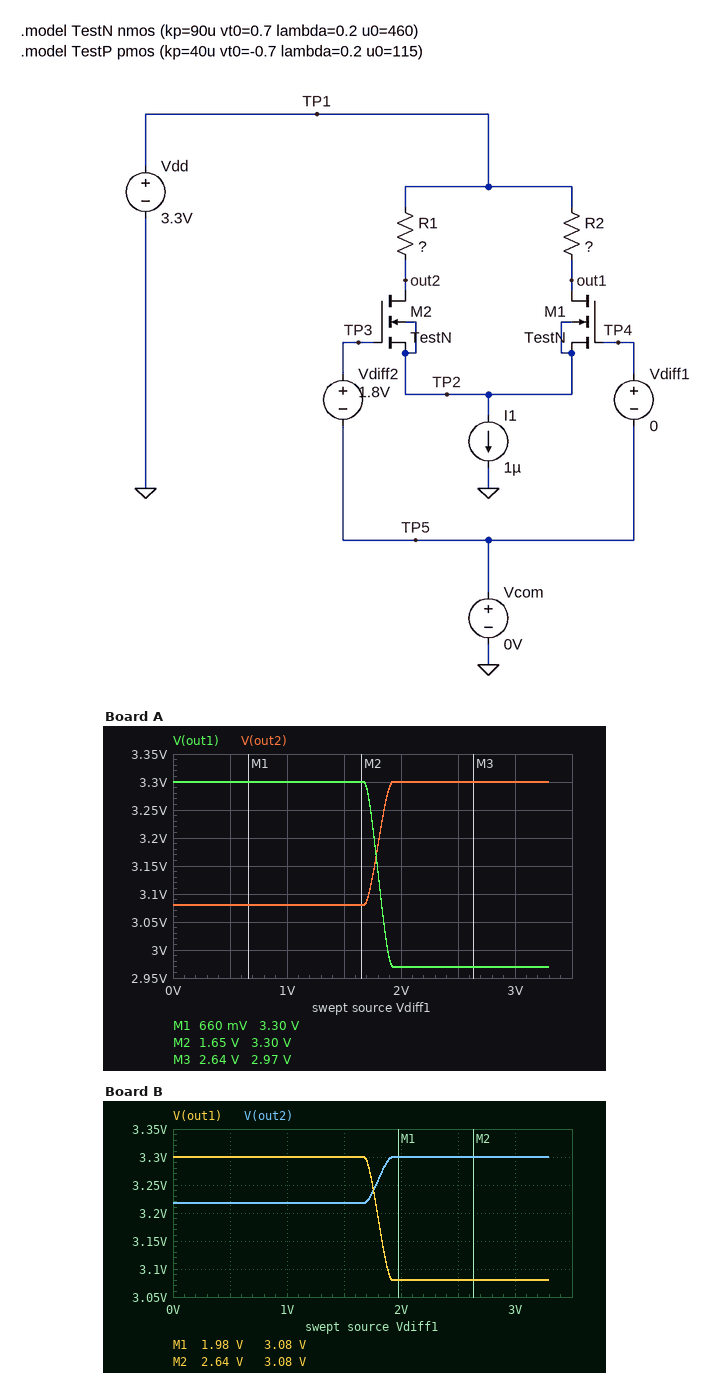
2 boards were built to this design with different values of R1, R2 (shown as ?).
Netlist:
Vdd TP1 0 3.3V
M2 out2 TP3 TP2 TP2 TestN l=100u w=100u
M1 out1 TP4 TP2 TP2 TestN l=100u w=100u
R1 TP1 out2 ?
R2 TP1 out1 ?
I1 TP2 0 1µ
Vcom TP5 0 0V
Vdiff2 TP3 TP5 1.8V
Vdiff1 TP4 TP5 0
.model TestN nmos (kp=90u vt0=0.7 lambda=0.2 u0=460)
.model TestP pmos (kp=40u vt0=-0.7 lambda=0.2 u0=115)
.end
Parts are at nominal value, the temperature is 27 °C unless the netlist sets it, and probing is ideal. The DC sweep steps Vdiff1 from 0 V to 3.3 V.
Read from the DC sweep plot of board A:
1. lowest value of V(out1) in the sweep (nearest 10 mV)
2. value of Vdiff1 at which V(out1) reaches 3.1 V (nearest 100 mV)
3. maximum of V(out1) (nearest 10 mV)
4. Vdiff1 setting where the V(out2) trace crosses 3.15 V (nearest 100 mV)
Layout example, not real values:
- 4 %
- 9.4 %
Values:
- 2.97 V
- 1.8 V
- 3.30 V
- 1.8 V
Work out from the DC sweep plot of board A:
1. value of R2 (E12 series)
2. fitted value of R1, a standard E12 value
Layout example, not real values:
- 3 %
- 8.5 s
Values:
- 330 kΩ
- 220 kΩ
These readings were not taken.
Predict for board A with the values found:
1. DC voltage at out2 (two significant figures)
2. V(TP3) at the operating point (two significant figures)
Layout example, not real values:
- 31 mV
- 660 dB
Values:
- 3.1 V
- 1.8 V
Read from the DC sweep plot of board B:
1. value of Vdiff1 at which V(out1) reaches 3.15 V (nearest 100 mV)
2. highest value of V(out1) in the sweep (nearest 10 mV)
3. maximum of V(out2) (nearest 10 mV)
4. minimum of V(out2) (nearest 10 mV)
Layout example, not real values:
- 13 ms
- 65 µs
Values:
- 1.8 V
- 3.30 V
- 3.30 V
- 3.22 V
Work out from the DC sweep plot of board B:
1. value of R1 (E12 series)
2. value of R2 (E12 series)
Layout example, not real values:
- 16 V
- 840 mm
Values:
- 82 kΩ
- 220 kΩ
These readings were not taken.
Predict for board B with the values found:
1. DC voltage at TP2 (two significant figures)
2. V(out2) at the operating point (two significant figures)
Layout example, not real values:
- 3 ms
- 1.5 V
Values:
- 980 mV
- 3.2 V
